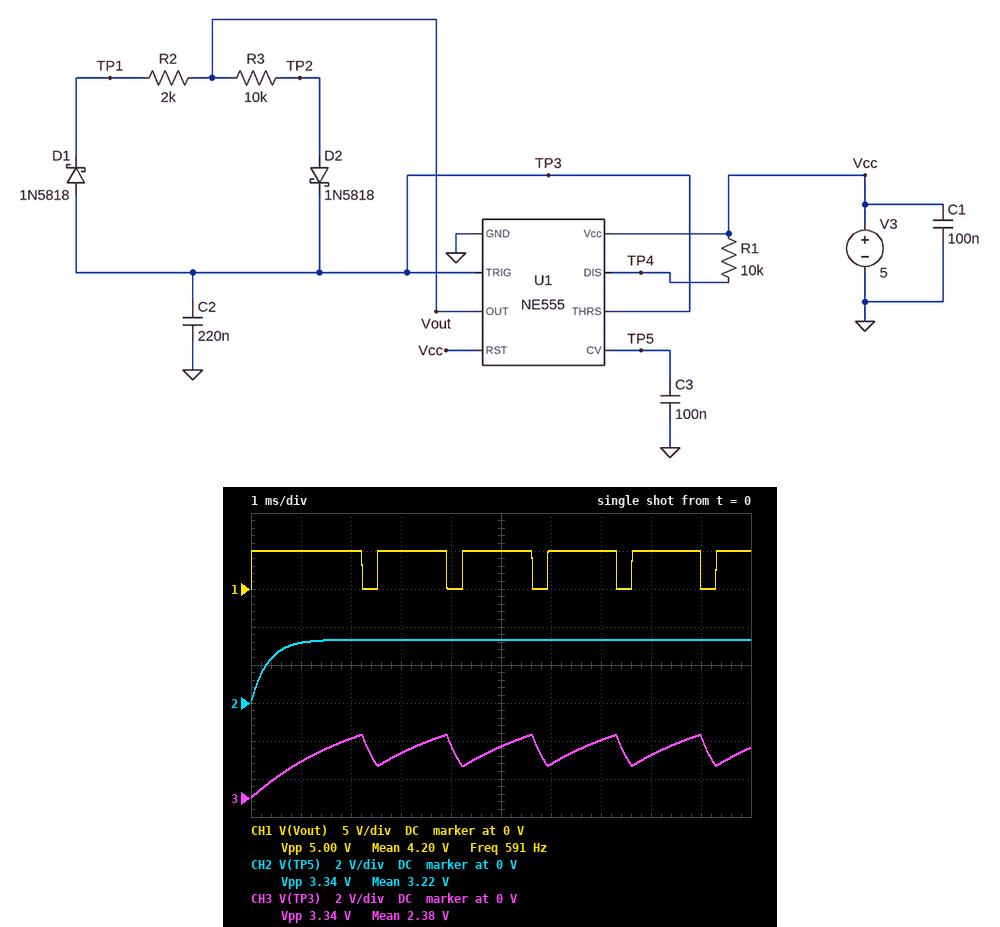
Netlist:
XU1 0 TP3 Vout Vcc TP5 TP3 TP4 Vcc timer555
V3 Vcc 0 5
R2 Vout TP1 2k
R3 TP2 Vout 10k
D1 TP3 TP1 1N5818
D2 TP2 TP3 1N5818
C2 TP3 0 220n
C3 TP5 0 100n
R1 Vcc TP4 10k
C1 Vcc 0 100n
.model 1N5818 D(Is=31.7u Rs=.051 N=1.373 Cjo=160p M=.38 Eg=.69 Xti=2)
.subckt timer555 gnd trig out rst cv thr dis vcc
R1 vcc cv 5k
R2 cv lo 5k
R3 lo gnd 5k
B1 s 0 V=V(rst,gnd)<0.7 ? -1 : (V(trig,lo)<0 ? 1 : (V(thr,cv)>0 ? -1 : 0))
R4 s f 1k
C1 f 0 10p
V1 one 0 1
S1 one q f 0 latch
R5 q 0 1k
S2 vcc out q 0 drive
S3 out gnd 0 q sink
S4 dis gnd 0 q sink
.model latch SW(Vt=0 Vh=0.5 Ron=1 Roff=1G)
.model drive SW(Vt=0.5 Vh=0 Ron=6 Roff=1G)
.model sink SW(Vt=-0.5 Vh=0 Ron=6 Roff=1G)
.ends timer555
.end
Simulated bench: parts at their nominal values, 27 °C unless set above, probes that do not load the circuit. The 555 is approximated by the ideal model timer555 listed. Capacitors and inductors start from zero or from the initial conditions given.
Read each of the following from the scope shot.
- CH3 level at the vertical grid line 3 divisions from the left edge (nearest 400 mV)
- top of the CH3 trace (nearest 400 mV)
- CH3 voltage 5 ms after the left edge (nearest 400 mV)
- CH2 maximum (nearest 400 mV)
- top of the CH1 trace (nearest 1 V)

2.4 V
3.2 V
2.8 V
3.2 V
5 V
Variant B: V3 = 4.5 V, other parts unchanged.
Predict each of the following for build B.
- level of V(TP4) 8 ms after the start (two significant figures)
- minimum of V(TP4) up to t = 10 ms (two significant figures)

4.5 V
2.7 mV
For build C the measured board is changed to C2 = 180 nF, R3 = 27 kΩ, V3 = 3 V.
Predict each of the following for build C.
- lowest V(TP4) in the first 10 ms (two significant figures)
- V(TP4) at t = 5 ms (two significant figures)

1.8 mV
3.0 V
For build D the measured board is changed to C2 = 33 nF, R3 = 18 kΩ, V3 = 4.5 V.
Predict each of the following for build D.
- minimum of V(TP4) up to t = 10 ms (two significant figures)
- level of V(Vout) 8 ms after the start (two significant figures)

2.7 mV
4.5 V
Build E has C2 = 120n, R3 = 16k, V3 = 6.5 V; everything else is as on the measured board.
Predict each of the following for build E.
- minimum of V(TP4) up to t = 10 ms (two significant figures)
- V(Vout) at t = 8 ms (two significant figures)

3.9 mV
6.5 V
